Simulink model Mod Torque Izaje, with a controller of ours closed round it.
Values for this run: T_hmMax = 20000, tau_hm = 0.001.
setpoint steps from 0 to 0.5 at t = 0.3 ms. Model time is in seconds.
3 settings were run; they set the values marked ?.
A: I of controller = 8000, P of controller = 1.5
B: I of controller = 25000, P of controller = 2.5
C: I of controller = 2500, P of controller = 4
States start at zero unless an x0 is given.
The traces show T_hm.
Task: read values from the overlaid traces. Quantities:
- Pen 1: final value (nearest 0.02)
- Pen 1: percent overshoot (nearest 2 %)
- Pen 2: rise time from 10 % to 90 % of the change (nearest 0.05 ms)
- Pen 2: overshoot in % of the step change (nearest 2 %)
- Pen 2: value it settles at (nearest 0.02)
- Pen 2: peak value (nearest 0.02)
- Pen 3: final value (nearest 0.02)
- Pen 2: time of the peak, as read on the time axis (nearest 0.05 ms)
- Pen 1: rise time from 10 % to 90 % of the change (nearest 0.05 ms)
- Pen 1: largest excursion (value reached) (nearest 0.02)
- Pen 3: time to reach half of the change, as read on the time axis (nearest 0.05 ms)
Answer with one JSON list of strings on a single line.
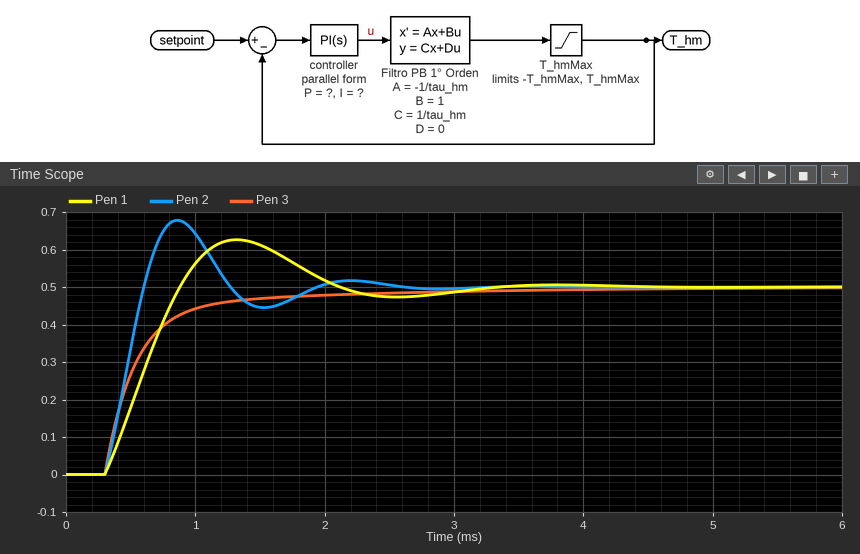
["0.50", "26 %", "0.25 ms", "36 %", "0.50", "0.68", "0.50", "0.85 ms", "0.45 ms", "0.62", "0.50 ms"]
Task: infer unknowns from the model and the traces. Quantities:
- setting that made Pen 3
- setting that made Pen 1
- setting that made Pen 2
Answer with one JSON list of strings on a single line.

["C", "A", "B"]
